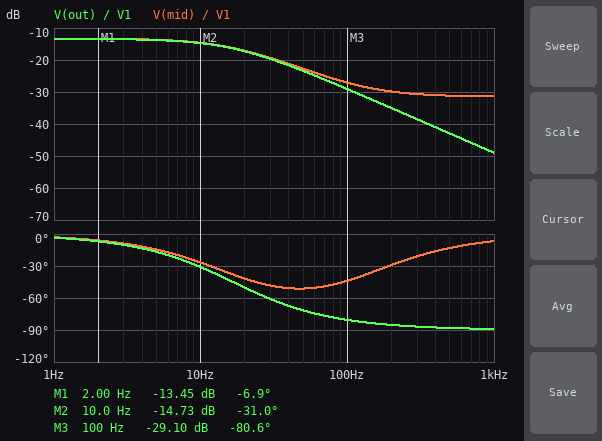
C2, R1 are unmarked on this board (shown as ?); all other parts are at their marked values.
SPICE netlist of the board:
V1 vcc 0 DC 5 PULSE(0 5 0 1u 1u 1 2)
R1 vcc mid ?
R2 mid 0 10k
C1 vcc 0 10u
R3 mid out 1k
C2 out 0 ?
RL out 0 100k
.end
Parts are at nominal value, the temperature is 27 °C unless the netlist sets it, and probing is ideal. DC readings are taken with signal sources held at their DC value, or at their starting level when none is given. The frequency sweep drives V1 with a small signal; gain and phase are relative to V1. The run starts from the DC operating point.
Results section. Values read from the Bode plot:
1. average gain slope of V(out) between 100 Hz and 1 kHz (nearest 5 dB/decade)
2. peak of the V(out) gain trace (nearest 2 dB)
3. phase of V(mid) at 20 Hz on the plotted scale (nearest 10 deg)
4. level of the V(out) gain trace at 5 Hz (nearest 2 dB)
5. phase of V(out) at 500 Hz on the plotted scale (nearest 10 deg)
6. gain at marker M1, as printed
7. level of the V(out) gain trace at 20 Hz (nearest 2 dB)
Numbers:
-20 dB/decade
-14 dB
-40 deg
-14 dB
-90 deg
-13.45 dB
-18 dB
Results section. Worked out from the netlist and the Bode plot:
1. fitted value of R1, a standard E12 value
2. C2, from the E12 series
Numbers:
33 kΩ
1.2 µF
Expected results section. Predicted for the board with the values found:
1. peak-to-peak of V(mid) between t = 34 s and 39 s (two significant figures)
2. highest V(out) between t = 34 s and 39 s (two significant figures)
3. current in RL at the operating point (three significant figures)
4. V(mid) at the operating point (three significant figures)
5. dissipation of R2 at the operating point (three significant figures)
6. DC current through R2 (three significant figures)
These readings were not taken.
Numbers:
1.1 V
1.1 V
10.7 µA
1.08 V
117 µW
108 µA
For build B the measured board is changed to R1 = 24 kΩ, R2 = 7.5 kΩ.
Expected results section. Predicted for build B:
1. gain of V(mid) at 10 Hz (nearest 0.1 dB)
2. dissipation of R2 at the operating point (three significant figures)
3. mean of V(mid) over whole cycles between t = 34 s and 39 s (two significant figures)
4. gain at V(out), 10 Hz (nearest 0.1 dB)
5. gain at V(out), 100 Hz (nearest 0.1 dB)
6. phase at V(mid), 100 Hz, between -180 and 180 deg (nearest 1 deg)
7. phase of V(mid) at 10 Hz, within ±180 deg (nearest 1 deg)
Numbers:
-13.8 dB
169 µW
560 mV
-13.9 dB
-26.7 dB
-41 deg
-21 deg
